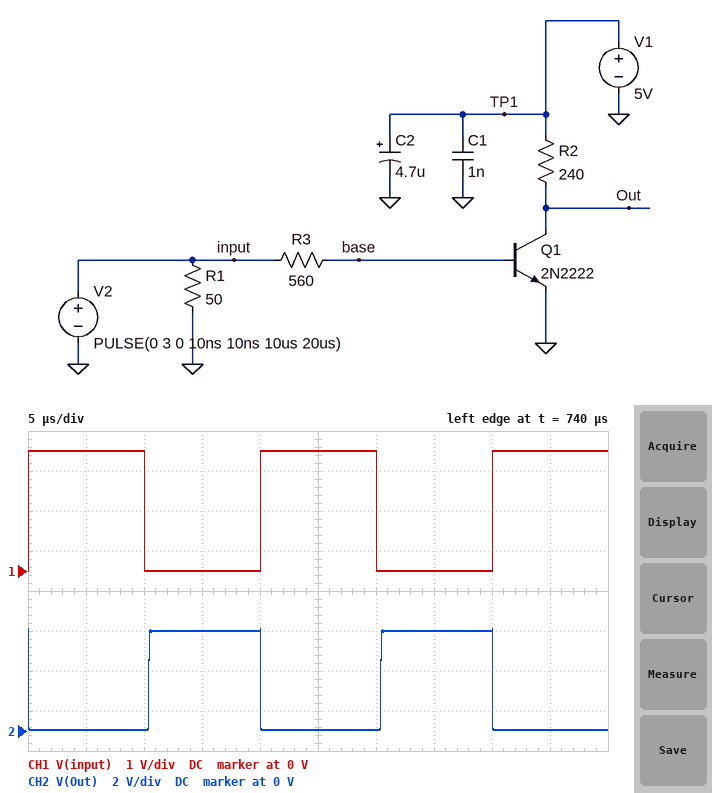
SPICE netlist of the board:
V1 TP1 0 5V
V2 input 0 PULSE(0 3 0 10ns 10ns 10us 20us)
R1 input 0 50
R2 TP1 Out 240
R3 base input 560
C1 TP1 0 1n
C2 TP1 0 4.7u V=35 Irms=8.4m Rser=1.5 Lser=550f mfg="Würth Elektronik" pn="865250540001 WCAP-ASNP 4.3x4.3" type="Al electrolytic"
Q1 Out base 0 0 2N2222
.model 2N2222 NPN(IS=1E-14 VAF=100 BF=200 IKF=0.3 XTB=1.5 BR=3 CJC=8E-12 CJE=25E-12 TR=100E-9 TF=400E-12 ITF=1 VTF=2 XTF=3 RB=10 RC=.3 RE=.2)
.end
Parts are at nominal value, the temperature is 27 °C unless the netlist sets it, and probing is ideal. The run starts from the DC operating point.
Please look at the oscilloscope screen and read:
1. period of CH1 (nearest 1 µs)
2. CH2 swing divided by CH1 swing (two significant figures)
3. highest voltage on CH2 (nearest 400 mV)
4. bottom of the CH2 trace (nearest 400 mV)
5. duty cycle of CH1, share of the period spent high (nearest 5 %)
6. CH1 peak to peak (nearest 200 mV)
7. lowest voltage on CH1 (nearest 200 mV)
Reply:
20 µs
1.7
5.2 V
0 V
50 %
3.0 V
0 V
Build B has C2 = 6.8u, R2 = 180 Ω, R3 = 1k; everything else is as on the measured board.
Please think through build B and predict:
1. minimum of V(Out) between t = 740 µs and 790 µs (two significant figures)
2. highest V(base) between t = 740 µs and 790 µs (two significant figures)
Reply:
60 mV
780 mV
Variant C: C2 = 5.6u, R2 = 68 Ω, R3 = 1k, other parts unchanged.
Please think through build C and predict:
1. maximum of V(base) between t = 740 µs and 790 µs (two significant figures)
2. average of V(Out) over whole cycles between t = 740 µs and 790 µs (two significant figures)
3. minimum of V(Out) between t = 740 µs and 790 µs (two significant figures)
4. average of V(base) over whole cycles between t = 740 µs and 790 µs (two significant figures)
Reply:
810 mV
2.5 V
110 mV
420 mV
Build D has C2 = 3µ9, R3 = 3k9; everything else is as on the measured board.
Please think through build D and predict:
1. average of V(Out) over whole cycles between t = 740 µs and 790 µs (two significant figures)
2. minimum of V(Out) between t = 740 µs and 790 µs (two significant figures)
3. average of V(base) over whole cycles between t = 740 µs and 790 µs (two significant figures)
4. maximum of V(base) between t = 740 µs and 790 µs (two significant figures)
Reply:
2.5 V
84 mV
390 mV
750 mV
